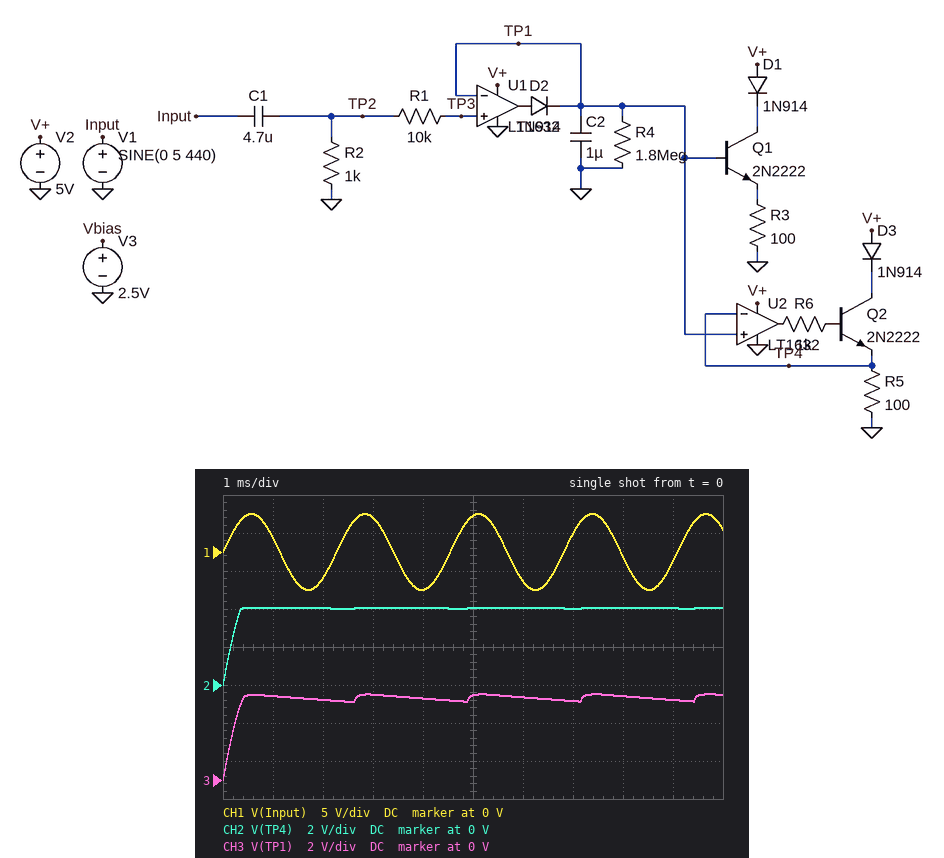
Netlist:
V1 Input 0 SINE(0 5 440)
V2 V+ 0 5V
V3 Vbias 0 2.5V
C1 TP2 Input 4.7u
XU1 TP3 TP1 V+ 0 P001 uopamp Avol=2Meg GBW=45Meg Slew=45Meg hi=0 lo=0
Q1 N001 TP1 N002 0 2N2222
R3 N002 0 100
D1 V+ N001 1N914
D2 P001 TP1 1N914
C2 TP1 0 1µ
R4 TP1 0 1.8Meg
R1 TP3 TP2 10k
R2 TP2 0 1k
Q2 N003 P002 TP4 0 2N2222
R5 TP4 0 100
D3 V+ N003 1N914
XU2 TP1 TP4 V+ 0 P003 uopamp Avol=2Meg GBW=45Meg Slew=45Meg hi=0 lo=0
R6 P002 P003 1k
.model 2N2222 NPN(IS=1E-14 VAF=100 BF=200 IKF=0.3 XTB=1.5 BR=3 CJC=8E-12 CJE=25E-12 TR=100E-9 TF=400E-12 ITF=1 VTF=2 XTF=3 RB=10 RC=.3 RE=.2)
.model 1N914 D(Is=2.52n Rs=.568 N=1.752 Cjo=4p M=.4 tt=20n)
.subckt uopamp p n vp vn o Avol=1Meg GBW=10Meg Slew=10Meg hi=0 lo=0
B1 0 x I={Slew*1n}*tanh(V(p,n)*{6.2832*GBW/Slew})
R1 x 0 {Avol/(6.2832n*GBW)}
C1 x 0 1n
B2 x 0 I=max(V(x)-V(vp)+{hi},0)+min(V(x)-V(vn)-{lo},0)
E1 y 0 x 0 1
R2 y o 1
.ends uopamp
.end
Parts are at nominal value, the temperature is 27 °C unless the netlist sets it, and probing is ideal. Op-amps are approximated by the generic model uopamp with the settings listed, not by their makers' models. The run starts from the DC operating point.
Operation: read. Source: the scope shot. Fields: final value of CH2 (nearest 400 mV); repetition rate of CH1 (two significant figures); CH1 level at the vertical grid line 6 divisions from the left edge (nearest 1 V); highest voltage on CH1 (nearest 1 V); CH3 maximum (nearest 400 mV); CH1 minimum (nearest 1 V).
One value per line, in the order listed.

4.0 V
440 Hz
-4 V
5 V
4.4 V
-5 V
